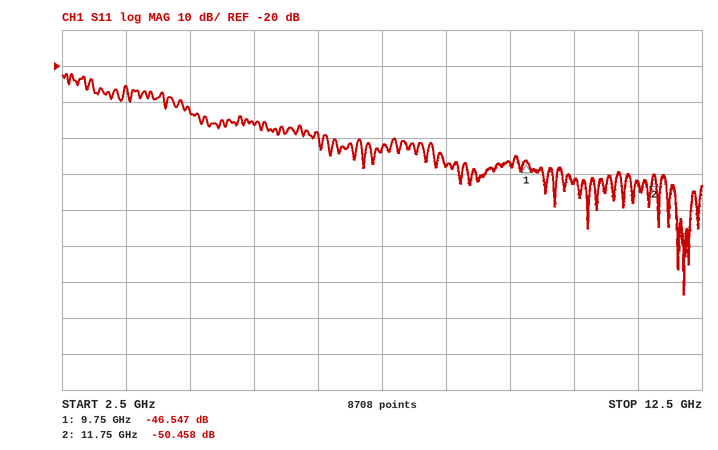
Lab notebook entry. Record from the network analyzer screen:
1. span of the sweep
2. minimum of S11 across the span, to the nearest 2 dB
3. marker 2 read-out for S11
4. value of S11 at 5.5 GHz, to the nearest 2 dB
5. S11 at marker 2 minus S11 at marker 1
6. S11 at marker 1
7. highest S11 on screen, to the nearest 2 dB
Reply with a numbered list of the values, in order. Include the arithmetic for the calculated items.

1. 10 GHz
2. -84 dB
3. -50.458 dB
4. -36 dB
5. -50.458 − (-46.547) = -3.911 dB
6. -46.547 dB
7. -22 dB
